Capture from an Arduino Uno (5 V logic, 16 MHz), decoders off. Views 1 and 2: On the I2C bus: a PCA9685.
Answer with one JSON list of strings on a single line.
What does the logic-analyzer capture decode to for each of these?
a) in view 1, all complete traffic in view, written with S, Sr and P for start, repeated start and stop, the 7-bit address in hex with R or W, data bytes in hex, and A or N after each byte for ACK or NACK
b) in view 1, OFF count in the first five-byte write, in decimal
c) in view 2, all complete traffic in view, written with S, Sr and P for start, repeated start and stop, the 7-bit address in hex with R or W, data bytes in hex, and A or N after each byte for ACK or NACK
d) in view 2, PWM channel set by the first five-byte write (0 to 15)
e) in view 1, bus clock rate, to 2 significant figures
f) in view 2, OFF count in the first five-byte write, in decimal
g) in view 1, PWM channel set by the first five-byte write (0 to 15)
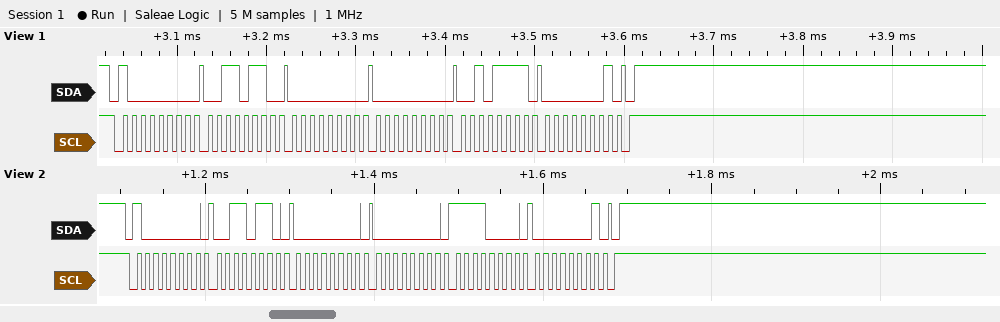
["S 40W A 36 A 00 A 00 A 2F A 01 A P", "303", "S 40W A 36 A 00 A 00 A F0 A 01 A P", "12", "100 kHz", "496", "12"]
